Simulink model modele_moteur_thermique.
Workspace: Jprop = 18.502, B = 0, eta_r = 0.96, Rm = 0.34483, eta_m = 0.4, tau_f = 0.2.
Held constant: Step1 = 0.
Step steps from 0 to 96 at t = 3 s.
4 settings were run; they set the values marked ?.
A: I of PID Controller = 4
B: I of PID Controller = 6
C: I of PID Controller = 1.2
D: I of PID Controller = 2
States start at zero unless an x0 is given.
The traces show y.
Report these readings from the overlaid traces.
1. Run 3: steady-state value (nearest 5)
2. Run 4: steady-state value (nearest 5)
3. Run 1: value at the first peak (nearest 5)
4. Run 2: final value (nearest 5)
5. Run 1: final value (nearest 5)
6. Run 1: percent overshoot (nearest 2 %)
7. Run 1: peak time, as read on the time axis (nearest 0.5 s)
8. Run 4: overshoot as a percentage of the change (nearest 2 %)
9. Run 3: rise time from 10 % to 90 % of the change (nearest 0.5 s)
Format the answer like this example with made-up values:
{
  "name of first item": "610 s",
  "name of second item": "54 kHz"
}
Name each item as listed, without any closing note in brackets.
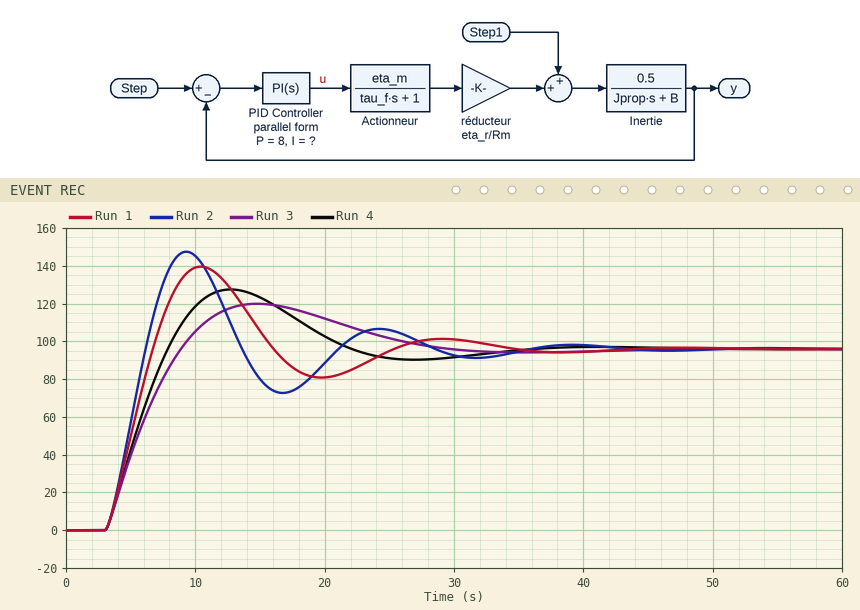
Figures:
{
  "Run 3: steady-state value": "95",
  "Run 4: steady-state value": "95",
  "Run 1: value at the first peak": "140",
  "Run 2: final value": "95",
  "Run 1: final value": "95",
  "Run 1: percent overshoot": "46 %",
  "Run 1: peak time, as read on the time axis": "10.5 s",
  "Run 4: overshoot as a percentage of the change": "32 %",
  "Run 3: rise time from 10 % to 90 % of the change": "4.5 s"
}
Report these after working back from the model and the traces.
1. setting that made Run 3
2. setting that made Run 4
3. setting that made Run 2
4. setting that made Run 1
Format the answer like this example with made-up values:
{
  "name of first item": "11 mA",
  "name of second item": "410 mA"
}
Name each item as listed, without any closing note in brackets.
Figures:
{
  "setting that made Run 3": "C",
  "setting that made Run 4": "D",
  "setting that made Run 2": "B",
  "setting that made Run 1": "A"
}
